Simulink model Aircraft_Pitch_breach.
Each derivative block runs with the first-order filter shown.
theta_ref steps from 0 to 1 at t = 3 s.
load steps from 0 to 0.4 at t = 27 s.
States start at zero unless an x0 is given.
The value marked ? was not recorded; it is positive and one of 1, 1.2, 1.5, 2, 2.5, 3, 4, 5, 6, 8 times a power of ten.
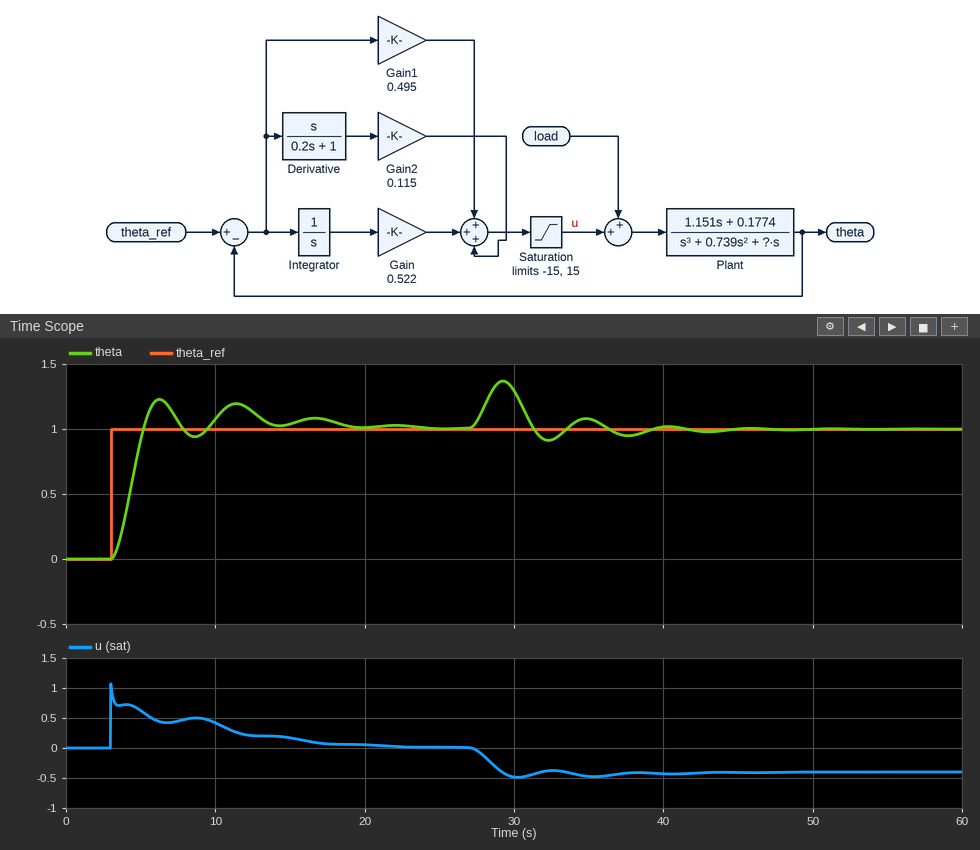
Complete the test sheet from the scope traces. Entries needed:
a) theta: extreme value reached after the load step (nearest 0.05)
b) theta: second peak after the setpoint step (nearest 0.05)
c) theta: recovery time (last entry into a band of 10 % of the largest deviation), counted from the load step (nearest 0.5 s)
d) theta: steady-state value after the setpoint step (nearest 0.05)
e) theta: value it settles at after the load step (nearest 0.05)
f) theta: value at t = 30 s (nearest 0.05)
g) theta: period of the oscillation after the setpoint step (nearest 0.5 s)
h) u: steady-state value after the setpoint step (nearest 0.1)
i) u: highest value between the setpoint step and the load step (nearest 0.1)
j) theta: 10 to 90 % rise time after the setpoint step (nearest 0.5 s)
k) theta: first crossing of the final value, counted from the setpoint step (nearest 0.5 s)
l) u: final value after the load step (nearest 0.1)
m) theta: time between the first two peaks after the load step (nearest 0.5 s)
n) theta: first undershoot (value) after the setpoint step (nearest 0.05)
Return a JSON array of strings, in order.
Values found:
["1.35", "1.20", "11.5 s", "1.00", "1.00", "1.30", "5.0 s", "0.0", "1.1", "1.5 s", "2.0 s", "-0.4", "5.5 s", "0.95"]
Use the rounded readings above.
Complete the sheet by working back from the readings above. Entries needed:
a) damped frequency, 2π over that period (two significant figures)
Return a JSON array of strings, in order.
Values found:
["1.3 rad/s"]
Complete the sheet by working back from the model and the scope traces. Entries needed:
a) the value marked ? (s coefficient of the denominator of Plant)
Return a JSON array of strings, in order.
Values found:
["1"]
